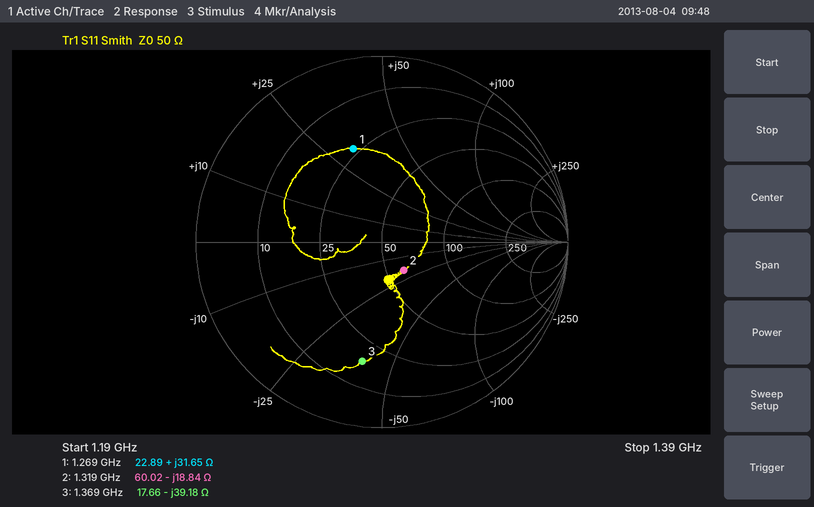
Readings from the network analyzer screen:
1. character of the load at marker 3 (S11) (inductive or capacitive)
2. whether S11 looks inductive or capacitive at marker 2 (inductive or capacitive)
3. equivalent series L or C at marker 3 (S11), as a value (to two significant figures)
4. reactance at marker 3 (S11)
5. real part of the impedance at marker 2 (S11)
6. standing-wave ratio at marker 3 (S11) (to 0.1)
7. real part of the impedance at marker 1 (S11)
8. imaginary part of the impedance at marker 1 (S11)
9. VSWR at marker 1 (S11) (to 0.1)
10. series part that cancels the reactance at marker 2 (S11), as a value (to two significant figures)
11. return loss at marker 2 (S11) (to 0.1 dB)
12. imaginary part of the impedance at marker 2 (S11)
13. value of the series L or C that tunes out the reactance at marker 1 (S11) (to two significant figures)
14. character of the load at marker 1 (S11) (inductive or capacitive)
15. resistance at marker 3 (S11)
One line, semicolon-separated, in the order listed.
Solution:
capacitive; capacitive; 3.0 pF; -39.18 Ω; 60.02 Ω; 4.7; 22.89 Ω; +31.65 Ω; 3.2; 2.3 nH; 14.4 dB; -18.84 Ω; 4.0 pF; inductive; 17.66 Ω
